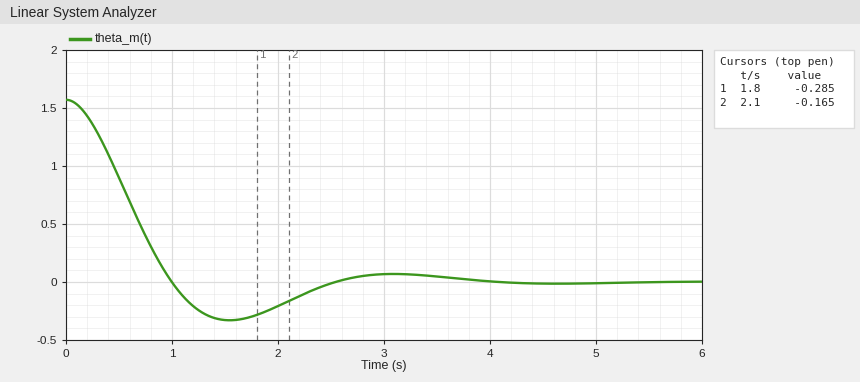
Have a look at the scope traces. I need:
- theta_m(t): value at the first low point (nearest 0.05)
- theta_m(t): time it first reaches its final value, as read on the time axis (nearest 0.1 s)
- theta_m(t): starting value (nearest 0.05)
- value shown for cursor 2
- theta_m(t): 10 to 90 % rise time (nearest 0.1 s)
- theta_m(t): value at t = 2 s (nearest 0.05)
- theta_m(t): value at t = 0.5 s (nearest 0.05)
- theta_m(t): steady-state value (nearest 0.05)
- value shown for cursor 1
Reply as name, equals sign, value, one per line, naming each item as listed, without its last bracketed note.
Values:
theta_m(t): value at the first low point = -0.35
theta_m(t): time it first reaches its final value, as read on the time axis = 1.0 s
theta_m(t): starting value = 1.55
value shown for cursor 2 = -0.165
theta_m(t): 10 to 90 % rise time = 0.7 s
theta_m(t): value at t = 2 s = -0.20
theta_m(t): value at t = 0.5 s = 0.90
theta_m(t): steady-state value = 0.00
value shown for cursor 1 = -0.285
